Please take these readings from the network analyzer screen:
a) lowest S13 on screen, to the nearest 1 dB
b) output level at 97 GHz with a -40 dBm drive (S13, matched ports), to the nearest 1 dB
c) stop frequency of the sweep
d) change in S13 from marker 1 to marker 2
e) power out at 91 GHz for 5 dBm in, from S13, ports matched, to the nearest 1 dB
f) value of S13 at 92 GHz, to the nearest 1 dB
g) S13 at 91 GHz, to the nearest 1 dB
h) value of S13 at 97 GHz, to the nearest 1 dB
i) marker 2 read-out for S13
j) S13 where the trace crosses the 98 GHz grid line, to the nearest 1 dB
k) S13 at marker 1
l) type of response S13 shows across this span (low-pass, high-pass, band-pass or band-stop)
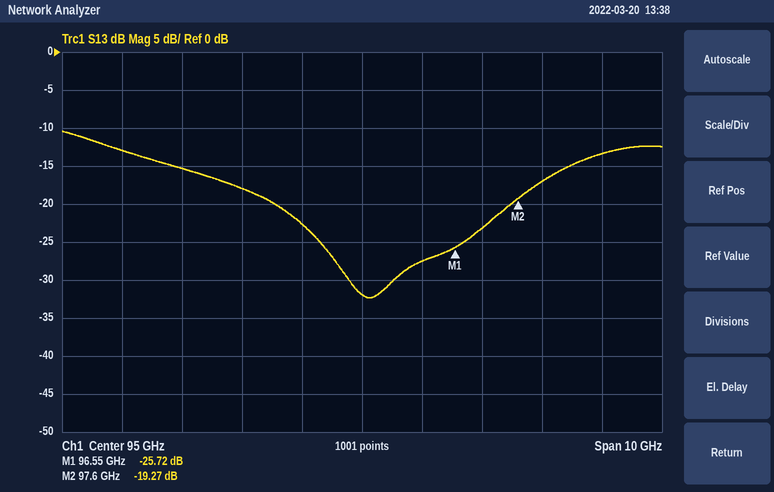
-32 dB
-63 dBm
100 GHz
6.45 dB
-8 dBm
-15 dB
-13 dB
-23 dB
-19.27 dB
-17 dB
-25.72 dB
band-stop
